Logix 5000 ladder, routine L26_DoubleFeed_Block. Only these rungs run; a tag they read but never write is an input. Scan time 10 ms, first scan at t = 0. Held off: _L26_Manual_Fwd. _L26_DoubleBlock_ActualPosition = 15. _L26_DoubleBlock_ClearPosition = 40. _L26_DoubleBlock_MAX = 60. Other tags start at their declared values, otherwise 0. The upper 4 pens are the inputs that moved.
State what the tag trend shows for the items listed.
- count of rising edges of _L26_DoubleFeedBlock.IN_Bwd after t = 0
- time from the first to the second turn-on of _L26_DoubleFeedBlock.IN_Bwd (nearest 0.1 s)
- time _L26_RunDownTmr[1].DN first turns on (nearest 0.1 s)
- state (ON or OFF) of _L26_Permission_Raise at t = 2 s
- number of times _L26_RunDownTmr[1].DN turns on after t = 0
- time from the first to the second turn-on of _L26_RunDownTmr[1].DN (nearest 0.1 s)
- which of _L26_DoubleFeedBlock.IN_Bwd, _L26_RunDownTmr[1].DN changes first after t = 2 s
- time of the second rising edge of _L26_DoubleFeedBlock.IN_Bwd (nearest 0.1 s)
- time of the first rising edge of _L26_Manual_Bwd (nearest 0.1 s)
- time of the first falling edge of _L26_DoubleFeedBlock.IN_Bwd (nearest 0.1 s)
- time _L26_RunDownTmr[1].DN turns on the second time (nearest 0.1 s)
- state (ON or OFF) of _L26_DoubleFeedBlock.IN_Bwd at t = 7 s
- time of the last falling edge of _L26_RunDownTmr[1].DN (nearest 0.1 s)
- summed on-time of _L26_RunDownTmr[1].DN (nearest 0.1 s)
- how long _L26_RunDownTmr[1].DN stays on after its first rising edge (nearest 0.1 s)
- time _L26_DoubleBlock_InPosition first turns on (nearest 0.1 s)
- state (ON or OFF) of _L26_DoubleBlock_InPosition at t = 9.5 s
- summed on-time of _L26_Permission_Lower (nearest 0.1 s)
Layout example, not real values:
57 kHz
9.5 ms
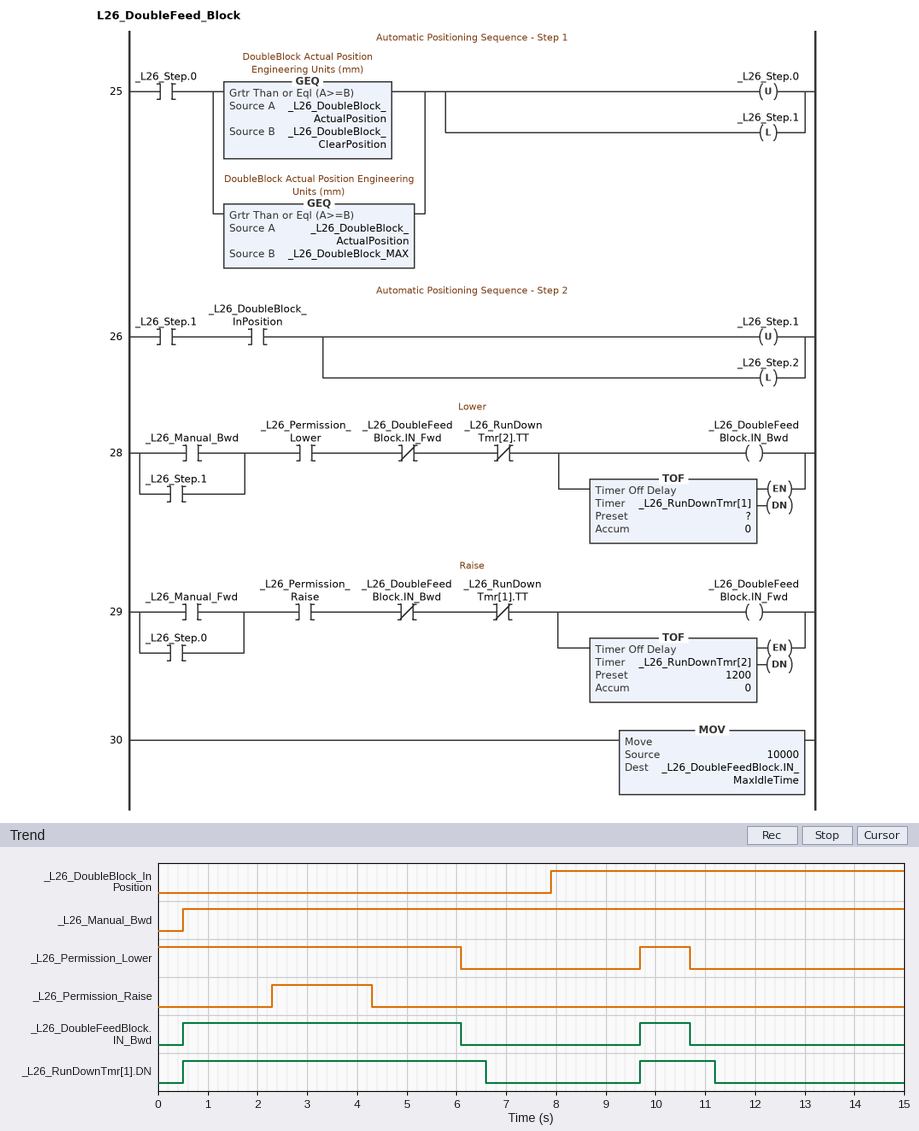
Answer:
2
9.2 s
0.5 s
OFF
2
9.2 s
_L26_DoubleFeedBlock.IN_Bwd
9.7 s
0.5 s
6.1 s
9.7 s
OFF
11.2 s
7.6 s
6.1 s
7.9 s
ON
7.1 s
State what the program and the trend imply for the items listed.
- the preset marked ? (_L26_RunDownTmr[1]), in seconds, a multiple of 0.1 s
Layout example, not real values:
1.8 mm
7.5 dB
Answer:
0.5 s
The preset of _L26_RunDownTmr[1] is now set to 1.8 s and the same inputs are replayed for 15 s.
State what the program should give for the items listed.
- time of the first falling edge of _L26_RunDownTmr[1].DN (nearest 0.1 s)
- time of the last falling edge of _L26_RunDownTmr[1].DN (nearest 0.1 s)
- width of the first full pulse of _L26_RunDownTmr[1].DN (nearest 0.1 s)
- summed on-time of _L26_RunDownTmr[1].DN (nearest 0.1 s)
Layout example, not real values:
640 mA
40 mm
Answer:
7.9 s
12.5 s
7.4 s
10.2 s
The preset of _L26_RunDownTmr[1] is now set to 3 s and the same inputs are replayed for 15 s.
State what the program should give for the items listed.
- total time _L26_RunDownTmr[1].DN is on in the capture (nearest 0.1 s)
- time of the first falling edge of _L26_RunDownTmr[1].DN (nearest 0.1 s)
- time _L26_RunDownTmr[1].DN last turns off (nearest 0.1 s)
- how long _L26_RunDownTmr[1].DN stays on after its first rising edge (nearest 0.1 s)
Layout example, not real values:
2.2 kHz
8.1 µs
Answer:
12.6 s
9.1 s
13.7 s
8.6 s
